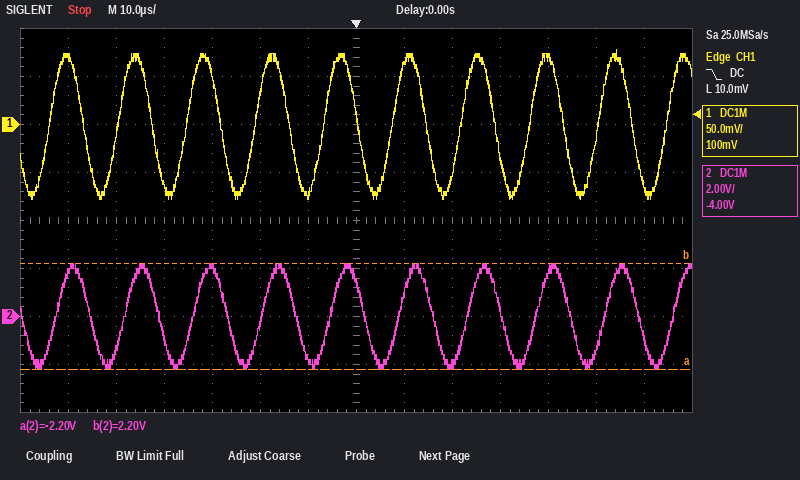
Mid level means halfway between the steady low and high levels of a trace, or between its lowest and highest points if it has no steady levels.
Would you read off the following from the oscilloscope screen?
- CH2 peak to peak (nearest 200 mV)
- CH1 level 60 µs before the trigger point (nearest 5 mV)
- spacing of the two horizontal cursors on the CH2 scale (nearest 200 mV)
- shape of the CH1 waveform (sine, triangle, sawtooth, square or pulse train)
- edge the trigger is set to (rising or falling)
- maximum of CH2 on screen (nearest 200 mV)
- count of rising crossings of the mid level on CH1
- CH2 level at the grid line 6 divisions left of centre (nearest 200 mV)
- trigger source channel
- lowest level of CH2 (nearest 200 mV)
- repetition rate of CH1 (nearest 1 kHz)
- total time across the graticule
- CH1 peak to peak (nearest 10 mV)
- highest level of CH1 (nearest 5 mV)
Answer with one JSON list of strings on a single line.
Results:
["4.4 V", "70 mV", "4.4 V", "sine", "falling", "2.2 V", "10", "1.8 V", "CH1", "-2.2 V", "70 kHz", "140 µs", "160 mV", "80 mV"]
